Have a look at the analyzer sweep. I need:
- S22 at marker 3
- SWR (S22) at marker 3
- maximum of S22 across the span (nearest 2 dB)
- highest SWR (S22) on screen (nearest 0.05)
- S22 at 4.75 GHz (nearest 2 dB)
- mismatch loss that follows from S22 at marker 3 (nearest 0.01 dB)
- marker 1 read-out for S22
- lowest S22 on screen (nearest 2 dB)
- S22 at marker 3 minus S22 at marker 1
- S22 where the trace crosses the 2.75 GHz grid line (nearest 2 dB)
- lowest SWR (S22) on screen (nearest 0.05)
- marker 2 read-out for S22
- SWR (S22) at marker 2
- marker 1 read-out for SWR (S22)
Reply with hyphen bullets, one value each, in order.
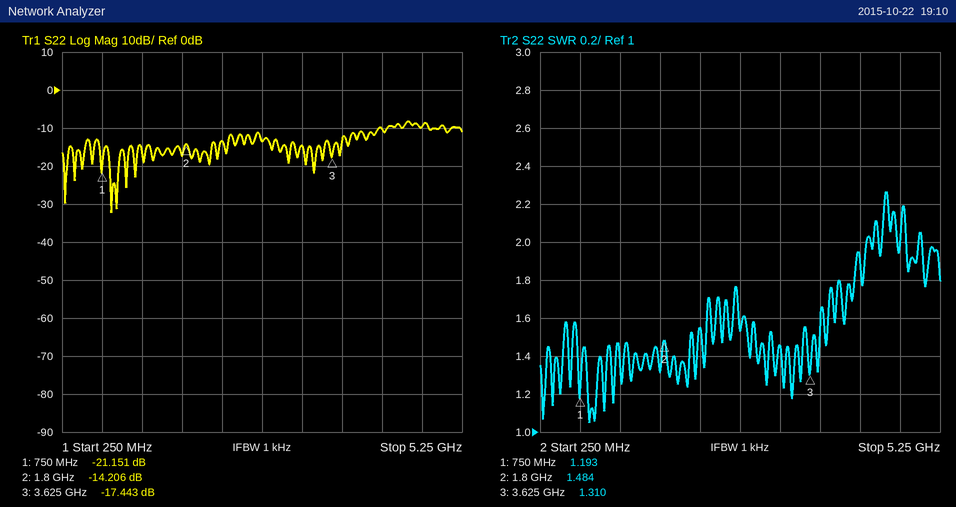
- -17.443 dB
- 1.310
- -8 dB
- 2.25
- -10 dB
- 0.08 dB
- -21.151 dB
- -32 dB
- 3.708 dB
- -14 dB
- 1.05
- -14.206 dB
- 1.484
- 1.193
